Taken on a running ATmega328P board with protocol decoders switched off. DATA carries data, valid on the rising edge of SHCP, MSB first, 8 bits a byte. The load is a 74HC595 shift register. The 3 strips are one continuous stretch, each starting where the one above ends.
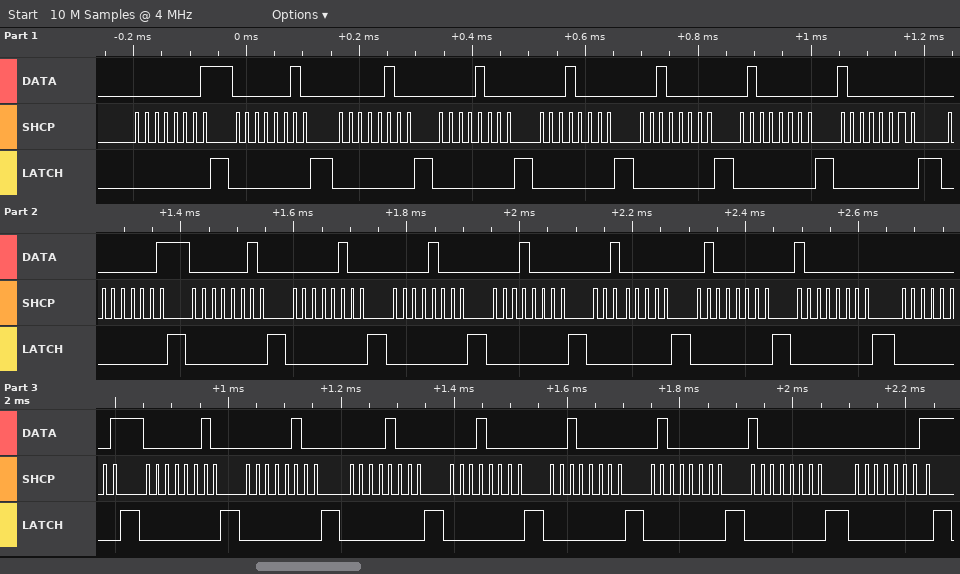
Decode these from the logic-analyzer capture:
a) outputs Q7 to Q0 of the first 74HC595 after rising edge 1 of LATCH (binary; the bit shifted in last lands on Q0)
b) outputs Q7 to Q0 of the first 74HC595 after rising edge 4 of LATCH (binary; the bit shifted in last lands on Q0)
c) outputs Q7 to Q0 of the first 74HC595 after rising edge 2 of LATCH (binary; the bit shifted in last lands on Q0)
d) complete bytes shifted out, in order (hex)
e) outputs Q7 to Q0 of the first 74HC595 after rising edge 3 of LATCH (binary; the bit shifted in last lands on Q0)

00000001
00001000
00000010
01 02 04 08 10 20 40 80 01 02 04 08 10 20 40 80 01 02 04 08 10 20 40 80 01
00000100
